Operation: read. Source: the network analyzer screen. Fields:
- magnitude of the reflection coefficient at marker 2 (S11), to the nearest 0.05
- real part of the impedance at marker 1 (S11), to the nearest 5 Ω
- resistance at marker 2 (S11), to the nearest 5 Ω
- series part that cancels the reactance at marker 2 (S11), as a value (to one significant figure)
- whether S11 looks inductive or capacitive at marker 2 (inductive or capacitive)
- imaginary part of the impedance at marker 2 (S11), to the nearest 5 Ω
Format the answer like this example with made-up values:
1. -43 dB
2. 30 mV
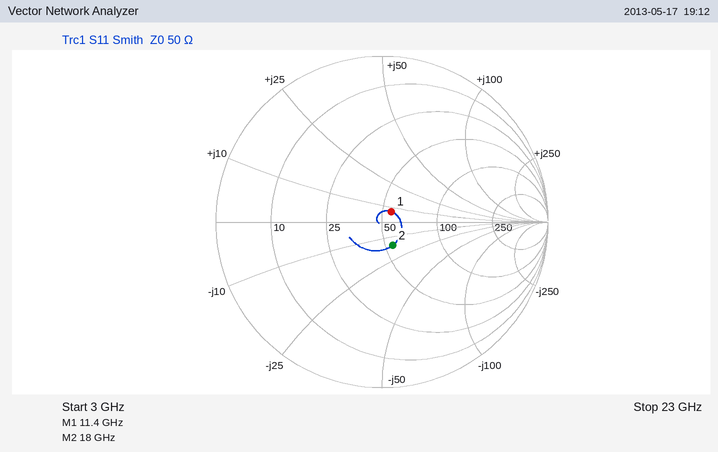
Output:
1. 0.15
2. 55 Ω
3. 55 Ω
4. 100 pH
5. capacitive
6. -15 Ω
